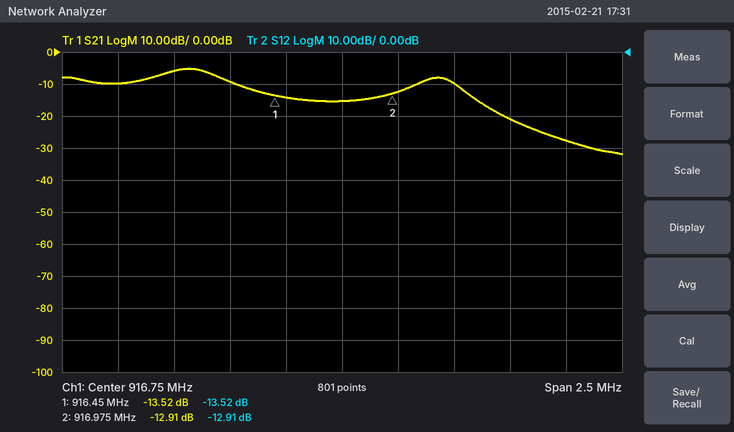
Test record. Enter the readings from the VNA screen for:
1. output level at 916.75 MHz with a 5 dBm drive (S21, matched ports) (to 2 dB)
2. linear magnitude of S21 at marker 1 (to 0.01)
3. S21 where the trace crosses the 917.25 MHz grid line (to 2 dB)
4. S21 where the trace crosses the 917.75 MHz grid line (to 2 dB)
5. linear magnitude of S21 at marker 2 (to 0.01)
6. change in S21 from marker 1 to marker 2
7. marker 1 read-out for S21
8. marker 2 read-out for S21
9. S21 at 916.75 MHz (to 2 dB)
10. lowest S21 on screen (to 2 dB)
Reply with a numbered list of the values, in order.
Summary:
1. -10 dBm
2. 0.21
3. -10 dB
4. -28 dB
5. 0.23
6. 0.61 dB
7. -13.52 dB
8. -12.91 dB
9. -16 dB
10. -32 dB
